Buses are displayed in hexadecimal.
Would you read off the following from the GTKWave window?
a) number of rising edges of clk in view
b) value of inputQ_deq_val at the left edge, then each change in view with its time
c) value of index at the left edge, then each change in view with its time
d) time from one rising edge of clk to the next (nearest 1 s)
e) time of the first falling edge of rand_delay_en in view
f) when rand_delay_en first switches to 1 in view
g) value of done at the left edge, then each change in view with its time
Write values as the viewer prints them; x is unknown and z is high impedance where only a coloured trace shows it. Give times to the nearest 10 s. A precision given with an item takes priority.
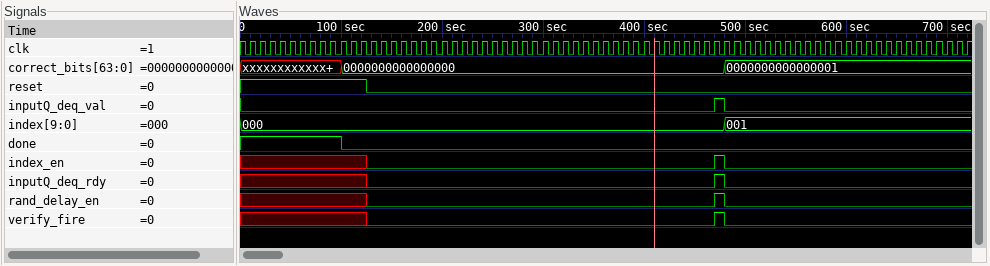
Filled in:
72
0, 1 at 470 s, 0 at 480 s
000, 001 at 480 s
10 s
480 s
470 s
1, 0 at 100 s
